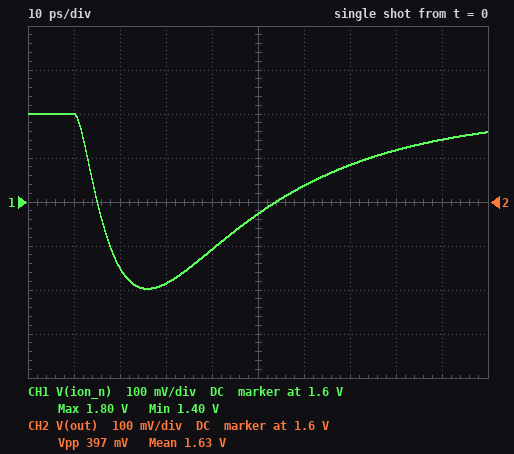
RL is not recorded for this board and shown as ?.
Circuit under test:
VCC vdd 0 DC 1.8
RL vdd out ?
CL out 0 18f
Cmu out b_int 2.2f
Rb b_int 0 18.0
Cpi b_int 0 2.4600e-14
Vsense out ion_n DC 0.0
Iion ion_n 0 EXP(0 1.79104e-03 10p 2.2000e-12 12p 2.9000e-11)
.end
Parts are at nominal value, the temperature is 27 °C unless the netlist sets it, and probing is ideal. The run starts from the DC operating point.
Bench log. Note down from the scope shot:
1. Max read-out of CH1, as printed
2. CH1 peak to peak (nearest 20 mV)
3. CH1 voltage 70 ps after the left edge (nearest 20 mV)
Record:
1.80 V
400 mV
1.68 V
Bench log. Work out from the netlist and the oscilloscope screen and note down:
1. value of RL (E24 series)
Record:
360 Ω
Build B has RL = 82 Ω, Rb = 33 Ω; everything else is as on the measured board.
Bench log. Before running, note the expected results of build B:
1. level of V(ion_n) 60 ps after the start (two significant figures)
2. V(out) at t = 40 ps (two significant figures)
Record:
1.8 V
1.7 V
